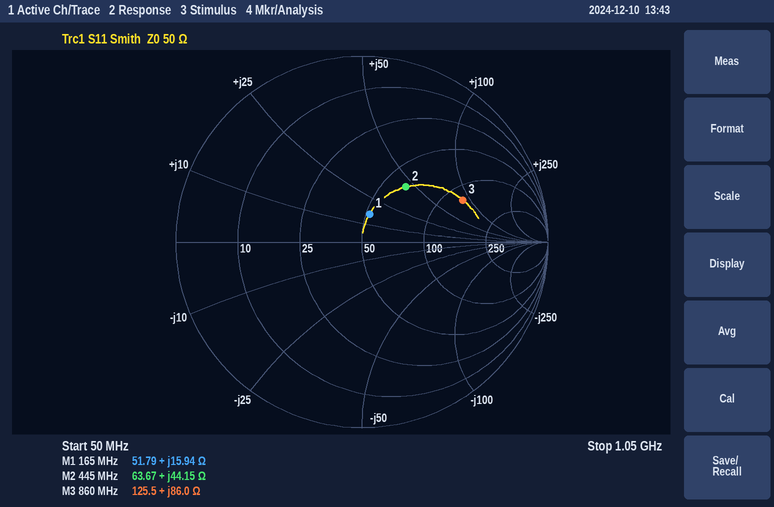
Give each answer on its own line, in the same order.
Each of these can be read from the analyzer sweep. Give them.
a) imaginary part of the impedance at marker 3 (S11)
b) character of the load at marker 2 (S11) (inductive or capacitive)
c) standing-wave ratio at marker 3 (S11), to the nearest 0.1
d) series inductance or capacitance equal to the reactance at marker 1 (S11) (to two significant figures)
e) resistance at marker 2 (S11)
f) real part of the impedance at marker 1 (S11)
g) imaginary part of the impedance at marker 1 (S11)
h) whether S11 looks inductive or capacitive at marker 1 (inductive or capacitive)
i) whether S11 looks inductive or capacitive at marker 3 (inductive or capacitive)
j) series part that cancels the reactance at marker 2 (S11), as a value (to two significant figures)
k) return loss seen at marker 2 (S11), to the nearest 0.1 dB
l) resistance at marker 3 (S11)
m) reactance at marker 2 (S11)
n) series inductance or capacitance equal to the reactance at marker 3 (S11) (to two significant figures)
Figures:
+86.0 Ω
inductive
3.8
15 nH
63.67 Ω
51.79 Ω
+15.94 Ω
inductive
inductive
8.1 pF
8.4 dB
125.5 Ω
+44.15 Ω
16 nH
